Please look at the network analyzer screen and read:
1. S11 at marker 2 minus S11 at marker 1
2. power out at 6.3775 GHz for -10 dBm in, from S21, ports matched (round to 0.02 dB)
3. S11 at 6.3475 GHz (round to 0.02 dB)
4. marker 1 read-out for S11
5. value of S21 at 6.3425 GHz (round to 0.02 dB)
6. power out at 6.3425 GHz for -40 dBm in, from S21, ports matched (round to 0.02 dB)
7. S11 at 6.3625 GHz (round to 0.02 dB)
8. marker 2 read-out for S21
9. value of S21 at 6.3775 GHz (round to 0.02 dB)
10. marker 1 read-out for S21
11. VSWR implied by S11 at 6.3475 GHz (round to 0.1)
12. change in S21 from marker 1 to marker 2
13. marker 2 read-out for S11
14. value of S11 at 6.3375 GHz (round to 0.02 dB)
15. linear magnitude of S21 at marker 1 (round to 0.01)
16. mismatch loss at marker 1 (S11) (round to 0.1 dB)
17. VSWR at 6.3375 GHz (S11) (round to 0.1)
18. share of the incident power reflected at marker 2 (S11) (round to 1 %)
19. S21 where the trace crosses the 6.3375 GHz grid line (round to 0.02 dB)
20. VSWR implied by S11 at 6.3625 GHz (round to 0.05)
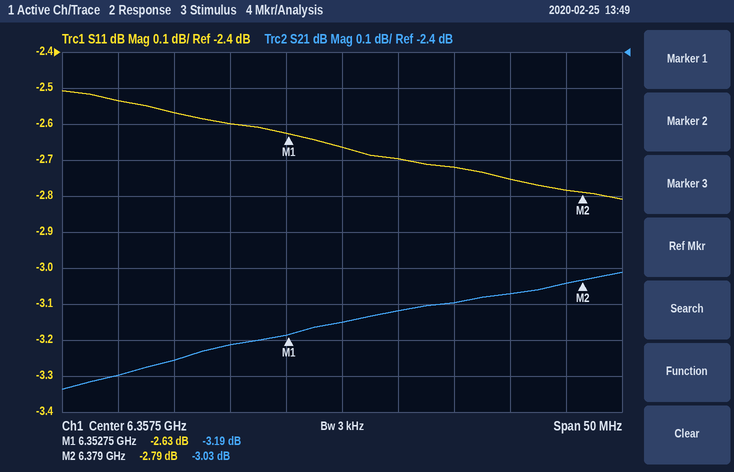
-0.16 dB
-13.04 dBm
-2.60 dB
-2.63 dB
-3.26 dB
-43.26 dBm
-2.70 dB
-3.03 dB
-3.04 dB
-3.19 dB
6.7
0.16 dB
-2.79 dB
-2.54 dB
0.69
3.4 dB
6.9
53 %
-3.30 dB
6.50
